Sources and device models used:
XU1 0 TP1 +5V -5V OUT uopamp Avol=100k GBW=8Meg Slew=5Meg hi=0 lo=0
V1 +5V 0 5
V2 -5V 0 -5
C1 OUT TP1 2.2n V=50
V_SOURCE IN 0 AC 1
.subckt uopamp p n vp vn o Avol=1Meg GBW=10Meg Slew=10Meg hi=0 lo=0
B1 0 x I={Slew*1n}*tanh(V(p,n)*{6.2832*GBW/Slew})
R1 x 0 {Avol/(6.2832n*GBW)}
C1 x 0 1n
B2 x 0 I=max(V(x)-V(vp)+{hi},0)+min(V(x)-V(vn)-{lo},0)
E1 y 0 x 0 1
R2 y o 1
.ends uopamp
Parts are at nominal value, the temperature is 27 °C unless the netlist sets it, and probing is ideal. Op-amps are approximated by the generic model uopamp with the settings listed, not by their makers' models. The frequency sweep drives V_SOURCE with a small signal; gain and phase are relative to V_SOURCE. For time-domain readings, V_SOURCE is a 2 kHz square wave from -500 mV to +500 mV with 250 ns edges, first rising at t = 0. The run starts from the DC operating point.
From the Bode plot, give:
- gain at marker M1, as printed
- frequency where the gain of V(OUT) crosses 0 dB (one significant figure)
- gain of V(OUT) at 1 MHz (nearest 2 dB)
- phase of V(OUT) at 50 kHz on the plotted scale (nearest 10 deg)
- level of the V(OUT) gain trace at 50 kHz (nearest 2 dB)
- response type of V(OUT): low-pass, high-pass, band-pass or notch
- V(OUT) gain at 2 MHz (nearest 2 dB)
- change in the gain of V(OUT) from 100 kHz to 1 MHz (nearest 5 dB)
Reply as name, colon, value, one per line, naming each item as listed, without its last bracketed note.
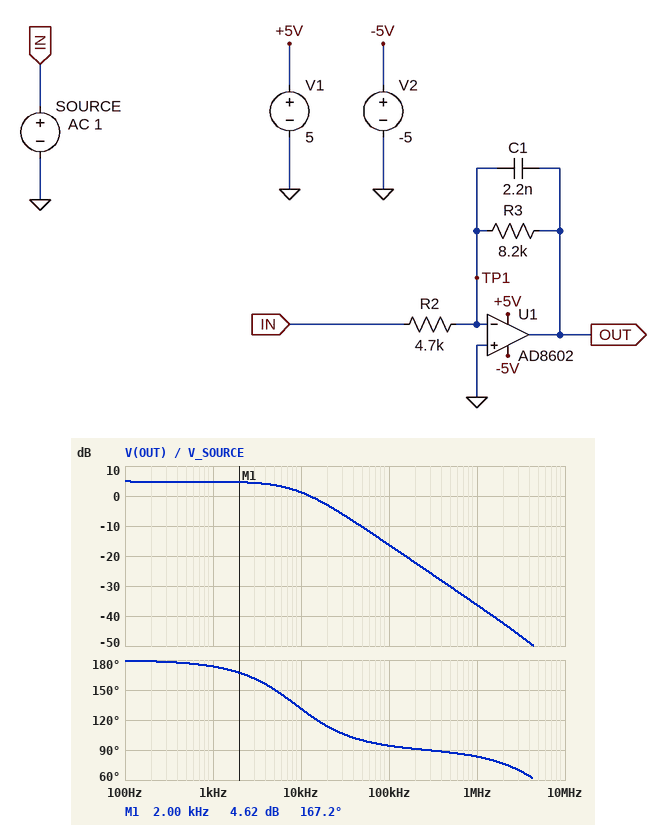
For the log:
gain at marker M1, as printed: 4.62 dB
frequency where the gain of V(OUT) crosses 0 dB: 10 kHz
gain of V(OUT) at 1 MHz: -36 dB
phase of V(OUT) at 50 kHz on the plotted scale: 100 deg
level of the V(OUT) gain trace at 50 kHz: -10 dB
response type of V(OUT): low-pass, high-pass, band-pass or notch: low-pass
V(OUT) gain at 2 MHz: -42 dB
change in the gain of V(OUT) from 100 kHz to 1 MHz: -20 dB
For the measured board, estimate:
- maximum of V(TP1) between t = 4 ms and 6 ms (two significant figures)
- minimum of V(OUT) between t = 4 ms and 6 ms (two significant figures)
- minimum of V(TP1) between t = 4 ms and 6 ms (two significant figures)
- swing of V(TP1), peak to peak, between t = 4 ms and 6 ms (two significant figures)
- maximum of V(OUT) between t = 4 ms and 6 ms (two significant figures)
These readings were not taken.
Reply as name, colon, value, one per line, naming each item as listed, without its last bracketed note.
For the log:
maximum of V(TP1) between t = 4 ms and 6 ms: 1.9 mV
minimum of V(OUT) between t = 4 ms and 6 ms: -870 mV
minimum of V(TP1) between t = 4 ms and 6 ms: -1.9 mV
swing of V(TP1), peak to peak, between t = 4 ms and 6 ms: 3.8 mV
maximum of V(OUT) between t = 4 ms and 6 ms: 870 mV
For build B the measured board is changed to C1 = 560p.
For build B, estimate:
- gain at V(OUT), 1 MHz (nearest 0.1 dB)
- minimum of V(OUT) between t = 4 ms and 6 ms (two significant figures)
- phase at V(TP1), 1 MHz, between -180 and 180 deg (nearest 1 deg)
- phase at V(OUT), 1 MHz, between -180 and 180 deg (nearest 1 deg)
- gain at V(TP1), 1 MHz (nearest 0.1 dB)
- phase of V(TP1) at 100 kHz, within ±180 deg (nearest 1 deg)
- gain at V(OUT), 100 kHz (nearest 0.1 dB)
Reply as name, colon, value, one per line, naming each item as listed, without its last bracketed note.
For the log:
gain at V(OUT), 1 MHz: -24.5 dB
minimum of V(OUT) between t = 4 ms and 6 ms: -870 mV
phase at V(TP1), 1 MHz, between -180 and 180 deg: -5 deg
phase at V(OUT), 1 MHz, between -180 and 180 deg: 85 deg
gain at V(TP1), 1 MHz: -42.6 dB
phase of V(TP1) at 100 kHz, within ±180 deg: 18 deg
gain at V(OUT), 100 kHz: -4.9 dB
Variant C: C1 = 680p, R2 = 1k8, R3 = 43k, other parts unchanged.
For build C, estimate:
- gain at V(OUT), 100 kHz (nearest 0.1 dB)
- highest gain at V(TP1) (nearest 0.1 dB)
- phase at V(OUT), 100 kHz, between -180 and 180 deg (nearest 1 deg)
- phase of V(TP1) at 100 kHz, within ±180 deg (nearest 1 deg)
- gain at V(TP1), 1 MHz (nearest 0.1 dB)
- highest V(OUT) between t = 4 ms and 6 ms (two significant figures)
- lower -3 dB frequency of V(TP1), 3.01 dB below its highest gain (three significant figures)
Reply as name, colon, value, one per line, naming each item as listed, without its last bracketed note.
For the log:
gain at V(OUT), 100 kHz: 2.1 dB
highest gain at V(TP1): -35.9 dB
phase at V(OUT), 100 kHz, between -180 and 180 deg: 92 deg
phase of V(TP1) at 100 kHz, within ±180 deg: 2 deg
gain at V(TP1), 1 MHz: -36.0 dB
highest V(OUT) between t = 4 ms and 6 ms: 5.0 V
lower -3 dB frequency of V(TP1), 3.01 dB below its highest gain: 5.35 kHz
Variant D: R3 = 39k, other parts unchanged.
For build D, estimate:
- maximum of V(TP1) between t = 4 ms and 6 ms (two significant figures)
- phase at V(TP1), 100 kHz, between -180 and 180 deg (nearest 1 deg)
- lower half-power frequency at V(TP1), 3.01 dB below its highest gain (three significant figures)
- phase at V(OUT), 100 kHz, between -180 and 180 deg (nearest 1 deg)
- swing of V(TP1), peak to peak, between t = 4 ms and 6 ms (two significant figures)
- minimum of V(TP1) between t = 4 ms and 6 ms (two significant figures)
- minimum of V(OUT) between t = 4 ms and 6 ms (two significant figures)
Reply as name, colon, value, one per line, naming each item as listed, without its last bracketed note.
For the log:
maximum of V(TP1) between t = 4 ms and 6 ms: 1.8 mV
phase at V(TP1), 100 kHz, between -180 and 180 deg: 0 deg
lower half-power frequency at V(TP1), 3.01 dB below its highest gain: 1.85 kHz
phase at V(OUT), 100 kHz, between -180 and 180 deg: 90 deg
swing of V(TP1), peak to peak, between t = 4 ms and 6 ms: 3.6 mV
minimum of V(TP1) between t = 4 ms and 6 ms: -1.8 mV
minimum of V(OUT) between t = 4 ms and 6 ms: -3.7 V
